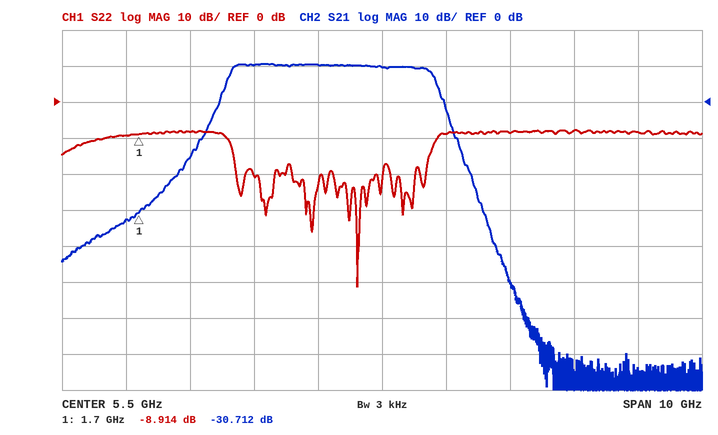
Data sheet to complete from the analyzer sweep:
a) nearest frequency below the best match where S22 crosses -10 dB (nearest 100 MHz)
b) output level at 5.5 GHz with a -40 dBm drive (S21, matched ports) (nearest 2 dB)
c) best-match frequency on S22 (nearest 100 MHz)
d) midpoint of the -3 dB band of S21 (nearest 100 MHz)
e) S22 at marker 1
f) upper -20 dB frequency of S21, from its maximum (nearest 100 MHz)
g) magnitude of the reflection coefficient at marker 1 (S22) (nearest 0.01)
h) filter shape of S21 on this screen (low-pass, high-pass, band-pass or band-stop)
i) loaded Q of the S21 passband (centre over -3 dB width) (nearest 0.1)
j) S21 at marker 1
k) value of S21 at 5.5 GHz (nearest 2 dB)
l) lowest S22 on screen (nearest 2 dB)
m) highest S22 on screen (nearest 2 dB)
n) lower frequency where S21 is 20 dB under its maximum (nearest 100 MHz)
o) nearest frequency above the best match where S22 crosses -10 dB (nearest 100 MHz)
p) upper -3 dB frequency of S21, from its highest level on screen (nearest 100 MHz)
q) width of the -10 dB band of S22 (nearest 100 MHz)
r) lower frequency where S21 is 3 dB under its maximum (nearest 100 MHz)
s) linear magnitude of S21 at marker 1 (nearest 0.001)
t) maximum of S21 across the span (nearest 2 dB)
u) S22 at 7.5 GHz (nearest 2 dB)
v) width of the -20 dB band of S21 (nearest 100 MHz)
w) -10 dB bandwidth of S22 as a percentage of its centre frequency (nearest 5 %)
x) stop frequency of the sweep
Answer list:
3.1 GHz
-30 dBm
5.1 GHz
4.7 GHz
-8.914 dB
6.6 GHz
0.36
band-pass
1.5
-30.712 dB
10 dB
-52 dB
-8 dB
2.7 GHz
6.4 GHz
6.3 GHz
3.3 GHz
3.1 GHz
0.029
10 dB
-8 dB
3.9 GHz
70 %
10.5 GHz
